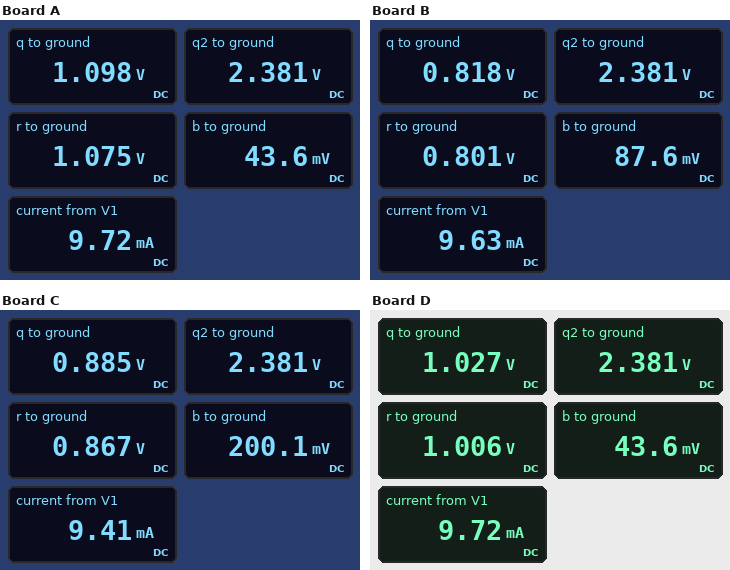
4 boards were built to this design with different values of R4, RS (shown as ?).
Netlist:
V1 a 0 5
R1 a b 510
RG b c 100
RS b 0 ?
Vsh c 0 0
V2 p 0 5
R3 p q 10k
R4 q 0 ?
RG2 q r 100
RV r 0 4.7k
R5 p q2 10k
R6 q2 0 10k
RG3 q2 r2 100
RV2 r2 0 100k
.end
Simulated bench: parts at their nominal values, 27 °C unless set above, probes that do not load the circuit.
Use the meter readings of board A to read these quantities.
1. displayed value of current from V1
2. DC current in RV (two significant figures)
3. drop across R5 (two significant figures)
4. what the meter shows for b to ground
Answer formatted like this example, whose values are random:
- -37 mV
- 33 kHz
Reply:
- 9.72 mA
- 230 µA
- 2.6 V
- 43.6 mV
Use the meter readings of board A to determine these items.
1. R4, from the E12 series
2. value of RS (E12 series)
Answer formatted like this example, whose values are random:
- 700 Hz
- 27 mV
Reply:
- 6.8 kΩ
- 4.7 Ω
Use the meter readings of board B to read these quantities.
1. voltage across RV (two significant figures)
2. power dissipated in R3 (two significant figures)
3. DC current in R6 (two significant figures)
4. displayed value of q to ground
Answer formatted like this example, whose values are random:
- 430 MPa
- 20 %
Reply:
- 800 mV
- 1.7 mW
- 240 µA
- 0.818 V
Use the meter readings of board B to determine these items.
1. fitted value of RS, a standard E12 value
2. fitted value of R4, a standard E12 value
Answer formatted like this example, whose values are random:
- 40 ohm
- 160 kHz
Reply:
- 10 Ω
- 3.3 kΩ
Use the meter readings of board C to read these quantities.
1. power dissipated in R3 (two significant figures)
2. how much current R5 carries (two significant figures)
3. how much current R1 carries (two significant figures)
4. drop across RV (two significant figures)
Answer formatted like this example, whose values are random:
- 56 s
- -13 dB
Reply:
- 1.7 mW
- 260 µA
- 9.4 mA
- 870 mV
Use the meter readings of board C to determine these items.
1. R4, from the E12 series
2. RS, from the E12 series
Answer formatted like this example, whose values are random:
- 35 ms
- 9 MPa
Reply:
- 3.9 kΩ
- 27 Ω
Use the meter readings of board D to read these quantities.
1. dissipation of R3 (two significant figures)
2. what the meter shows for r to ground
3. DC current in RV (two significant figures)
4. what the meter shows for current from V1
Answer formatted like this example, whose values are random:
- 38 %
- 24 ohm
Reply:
- 1.6 mW
- 1.006 V
- 210 µA
- 9.72 mA
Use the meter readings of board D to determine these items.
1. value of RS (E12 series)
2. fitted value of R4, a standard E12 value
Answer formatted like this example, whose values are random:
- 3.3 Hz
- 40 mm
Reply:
- 4.7 Ω
- 5.6 kΩ
